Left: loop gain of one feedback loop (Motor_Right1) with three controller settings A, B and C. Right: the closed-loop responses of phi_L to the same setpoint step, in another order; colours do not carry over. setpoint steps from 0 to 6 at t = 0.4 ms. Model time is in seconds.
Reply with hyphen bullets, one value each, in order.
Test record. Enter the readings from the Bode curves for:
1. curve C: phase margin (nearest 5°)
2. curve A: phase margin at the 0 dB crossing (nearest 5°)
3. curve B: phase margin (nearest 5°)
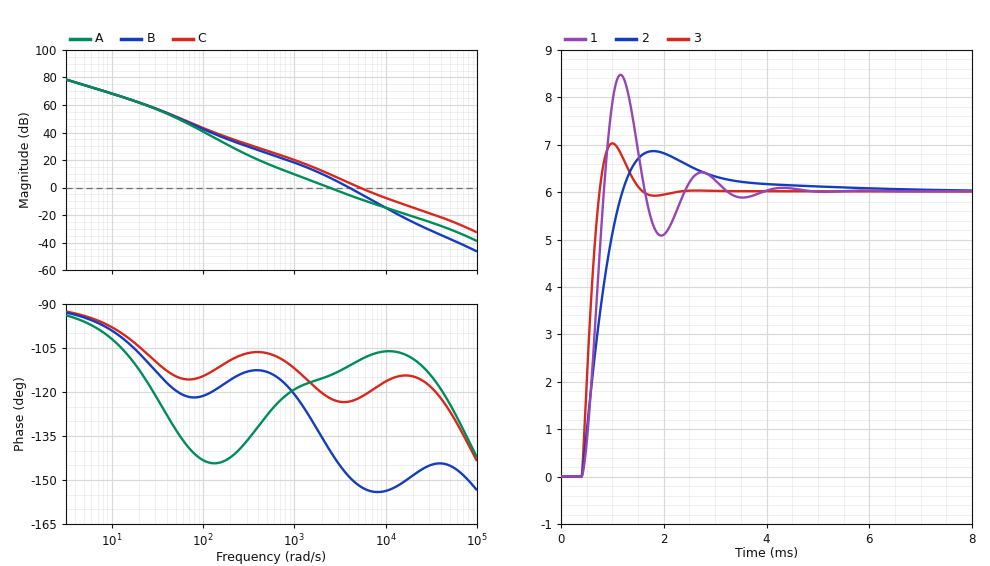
- 60°
- 65°
- 30°
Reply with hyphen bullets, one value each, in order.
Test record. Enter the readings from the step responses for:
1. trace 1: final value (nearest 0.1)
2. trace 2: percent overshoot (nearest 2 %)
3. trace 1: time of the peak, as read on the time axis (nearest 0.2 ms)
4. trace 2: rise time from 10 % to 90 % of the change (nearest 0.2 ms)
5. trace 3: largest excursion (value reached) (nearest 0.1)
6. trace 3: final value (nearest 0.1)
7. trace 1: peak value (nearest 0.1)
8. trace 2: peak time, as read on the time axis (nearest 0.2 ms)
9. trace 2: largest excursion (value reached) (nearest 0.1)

- 6.0
- 14 %
- 1.2 ms
- 0.6 ms
- 7.0
- 6.0
- 8.5
- 1.8 ms
- 6.9
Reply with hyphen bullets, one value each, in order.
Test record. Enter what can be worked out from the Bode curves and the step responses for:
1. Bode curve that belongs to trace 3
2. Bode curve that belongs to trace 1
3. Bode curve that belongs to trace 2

- C
- B
- A
